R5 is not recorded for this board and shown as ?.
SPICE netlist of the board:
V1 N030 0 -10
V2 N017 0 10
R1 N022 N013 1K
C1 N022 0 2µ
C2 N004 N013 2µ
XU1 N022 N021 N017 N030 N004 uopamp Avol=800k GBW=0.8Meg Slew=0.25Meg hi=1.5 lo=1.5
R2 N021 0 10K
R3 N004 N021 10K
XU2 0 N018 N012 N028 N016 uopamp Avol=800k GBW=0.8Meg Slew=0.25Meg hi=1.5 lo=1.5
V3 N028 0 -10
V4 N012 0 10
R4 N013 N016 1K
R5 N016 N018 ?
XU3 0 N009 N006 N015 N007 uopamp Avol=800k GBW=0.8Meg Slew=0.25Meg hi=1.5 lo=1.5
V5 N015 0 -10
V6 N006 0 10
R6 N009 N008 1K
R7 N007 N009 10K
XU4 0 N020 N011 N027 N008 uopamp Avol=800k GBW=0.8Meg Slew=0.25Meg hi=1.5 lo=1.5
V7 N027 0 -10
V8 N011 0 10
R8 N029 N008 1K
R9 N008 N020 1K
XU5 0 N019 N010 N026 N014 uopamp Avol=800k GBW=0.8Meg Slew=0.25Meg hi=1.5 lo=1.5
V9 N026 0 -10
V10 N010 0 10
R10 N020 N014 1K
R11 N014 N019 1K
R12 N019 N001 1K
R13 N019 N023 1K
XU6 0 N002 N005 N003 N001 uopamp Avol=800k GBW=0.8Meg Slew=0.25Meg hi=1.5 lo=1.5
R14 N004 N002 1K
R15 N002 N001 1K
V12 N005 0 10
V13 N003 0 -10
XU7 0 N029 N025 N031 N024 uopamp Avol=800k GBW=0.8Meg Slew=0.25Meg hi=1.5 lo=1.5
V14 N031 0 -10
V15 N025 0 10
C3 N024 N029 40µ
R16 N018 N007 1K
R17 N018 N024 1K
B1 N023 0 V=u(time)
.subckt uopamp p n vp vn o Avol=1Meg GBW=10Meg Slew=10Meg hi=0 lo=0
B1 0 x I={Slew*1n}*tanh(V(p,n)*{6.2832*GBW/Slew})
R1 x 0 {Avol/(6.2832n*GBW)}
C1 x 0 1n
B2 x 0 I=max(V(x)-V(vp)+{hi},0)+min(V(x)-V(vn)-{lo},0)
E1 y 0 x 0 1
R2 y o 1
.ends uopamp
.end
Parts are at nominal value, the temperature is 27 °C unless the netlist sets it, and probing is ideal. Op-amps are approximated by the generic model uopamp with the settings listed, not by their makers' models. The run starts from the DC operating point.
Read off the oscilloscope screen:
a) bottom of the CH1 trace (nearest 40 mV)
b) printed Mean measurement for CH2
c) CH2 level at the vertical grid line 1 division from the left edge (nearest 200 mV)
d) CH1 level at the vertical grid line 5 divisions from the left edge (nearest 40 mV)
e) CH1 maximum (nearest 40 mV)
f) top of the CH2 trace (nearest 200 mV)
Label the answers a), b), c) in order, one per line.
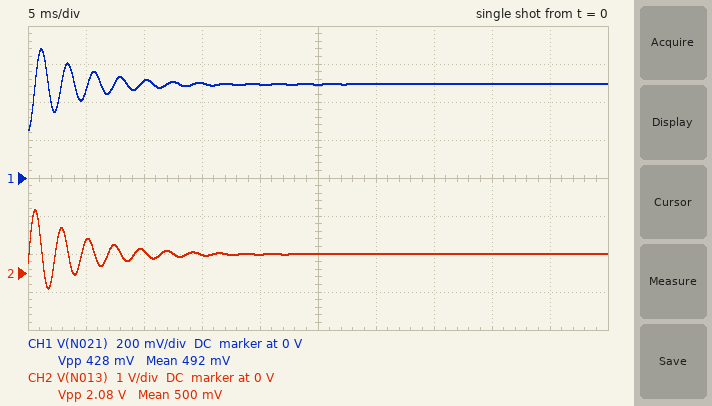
a) 240 mV
b) 500 mV
c) 800 mV
d) 480 mV
e) 680 mV
f) 1.6 V
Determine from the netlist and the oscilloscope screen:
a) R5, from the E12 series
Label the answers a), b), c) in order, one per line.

a) 1.5 kΩ
